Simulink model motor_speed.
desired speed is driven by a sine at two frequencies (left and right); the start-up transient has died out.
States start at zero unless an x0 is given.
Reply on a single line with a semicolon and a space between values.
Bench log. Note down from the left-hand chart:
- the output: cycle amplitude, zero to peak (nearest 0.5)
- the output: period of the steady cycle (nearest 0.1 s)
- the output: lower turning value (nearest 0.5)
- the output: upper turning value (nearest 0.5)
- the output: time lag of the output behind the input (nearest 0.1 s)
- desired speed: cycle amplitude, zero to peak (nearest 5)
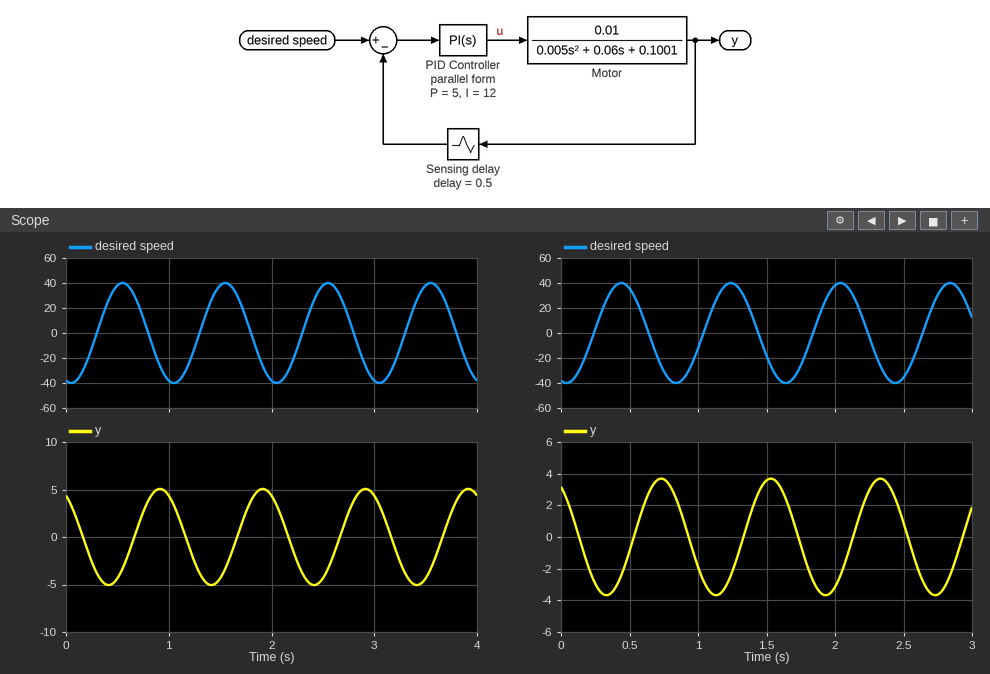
5.0; 1.0 s; -5.0; 5.0; 0.4 s; 40
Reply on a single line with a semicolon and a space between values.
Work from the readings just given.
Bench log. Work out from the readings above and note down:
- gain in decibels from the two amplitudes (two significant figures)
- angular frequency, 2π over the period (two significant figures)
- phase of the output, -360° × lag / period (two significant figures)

-18 dB; 6.3 rad/s; -140°
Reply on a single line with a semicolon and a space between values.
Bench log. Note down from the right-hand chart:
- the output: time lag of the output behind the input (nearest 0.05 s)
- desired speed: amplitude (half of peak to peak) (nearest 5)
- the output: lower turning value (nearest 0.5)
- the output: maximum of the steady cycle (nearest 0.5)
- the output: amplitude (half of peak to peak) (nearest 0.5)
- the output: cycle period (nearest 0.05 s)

0.30 s; 40; -3.5; 3.5; 3.5; 0.80 s
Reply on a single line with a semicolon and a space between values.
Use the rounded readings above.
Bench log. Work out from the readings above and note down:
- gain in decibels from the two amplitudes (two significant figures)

-21 dB
